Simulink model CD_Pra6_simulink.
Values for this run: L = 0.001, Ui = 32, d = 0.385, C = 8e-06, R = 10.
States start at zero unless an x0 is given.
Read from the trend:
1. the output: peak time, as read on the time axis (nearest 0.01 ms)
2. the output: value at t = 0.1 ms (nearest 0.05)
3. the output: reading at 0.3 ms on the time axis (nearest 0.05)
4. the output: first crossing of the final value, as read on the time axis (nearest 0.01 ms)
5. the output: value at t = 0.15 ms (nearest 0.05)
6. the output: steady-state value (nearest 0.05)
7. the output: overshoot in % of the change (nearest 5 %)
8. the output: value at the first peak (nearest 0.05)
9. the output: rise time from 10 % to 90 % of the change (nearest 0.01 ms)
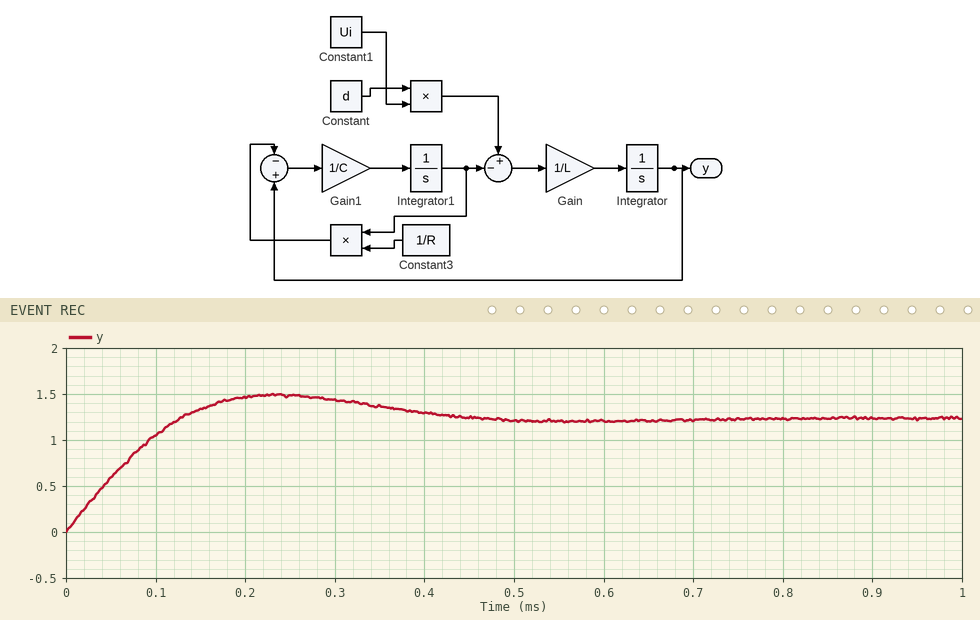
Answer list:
0.23 ms
1.05
1.45
0.13 ms
1.35
1.25
20 %
1.50
0.10 ms
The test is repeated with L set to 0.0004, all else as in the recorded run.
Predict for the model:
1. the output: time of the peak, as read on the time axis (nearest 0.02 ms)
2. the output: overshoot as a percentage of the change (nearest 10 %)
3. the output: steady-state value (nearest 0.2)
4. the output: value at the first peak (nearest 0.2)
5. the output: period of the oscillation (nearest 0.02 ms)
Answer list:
0.12 ms
70 %
1.2
2.0
0.38 ms
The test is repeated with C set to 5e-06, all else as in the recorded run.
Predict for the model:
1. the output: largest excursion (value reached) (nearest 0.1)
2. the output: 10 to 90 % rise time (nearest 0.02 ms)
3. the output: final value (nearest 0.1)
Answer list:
1.3
0.12 ms
1.2
